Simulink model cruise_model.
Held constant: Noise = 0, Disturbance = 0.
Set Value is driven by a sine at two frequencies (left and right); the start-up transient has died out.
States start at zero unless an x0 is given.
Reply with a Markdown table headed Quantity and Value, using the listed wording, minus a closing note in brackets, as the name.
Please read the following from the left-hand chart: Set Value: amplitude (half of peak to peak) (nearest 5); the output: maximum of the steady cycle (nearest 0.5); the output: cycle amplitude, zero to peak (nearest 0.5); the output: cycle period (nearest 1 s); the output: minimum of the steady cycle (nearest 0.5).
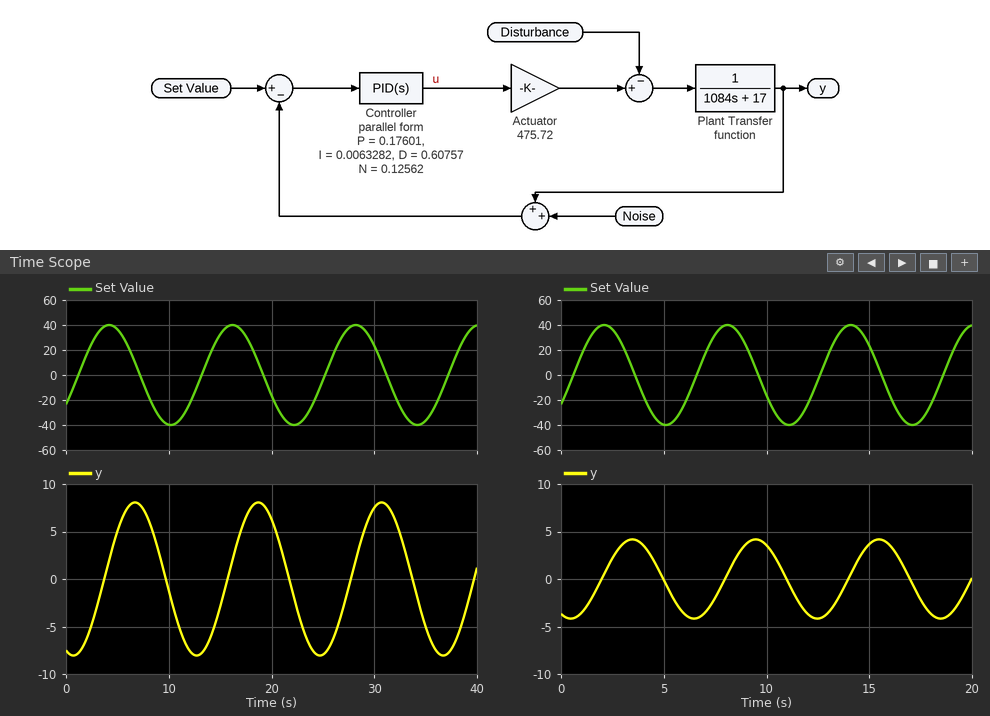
| Quantity | Value |
|---|---|
| Set Value: amplitude (half of peak to peak) | 40 |
| the output: maximum of the steady cycle | 8.0 |
| the output: cycle amplitude, zero to peak | 8.0 |
| the output: cycle period | 12 s |
| the output: minimum of the steady cycle | -8.0 |
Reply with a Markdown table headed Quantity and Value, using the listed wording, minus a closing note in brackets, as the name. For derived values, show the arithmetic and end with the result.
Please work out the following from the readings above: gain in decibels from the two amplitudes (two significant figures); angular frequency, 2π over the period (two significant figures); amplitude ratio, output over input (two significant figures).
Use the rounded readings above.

| Quantity | Value |
|---|---|
| gain in decibels from the two amplitudes | 20 log10(8 / 40) = -14 dB |
| angular frequency, 2π over the period | 2π / 12 = 0.52 rad/s |
| amplitude ratio, output over input | 8 / 40 = 0.20 |
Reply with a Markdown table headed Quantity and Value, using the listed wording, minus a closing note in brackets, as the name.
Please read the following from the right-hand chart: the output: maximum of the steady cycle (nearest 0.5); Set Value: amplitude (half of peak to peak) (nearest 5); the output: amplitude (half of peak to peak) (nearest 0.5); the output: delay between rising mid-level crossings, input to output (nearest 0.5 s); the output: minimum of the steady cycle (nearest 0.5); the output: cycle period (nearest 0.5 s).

| Quantity | Value |
|---|---|
| the output: maximum of the steady cycle | 4.0 |
| Set Value: amplitude (half of peak to peak) | 40 |
| the output: amplitude (half of peak to peak) | 4.0 |
| the output: delay between rising mid-level crossings, input to output | 1.5 s |
| the output: minimum of the steady cycle | -4.0 |
| the output: cycle period | 6.0 s |
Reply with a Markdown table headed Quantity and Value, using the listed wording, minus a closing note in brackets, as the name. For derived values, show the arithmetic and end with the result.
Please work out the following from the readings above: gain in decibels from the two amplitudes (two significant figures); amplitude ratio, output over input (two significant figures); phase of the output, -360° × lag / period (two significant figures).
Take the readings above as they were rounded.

| Quantity | Value |
|---|---|
| gain in decibels from the two amplitudes | 20 log10(4 / 40) = -20 dB |
| amplitude ratio, output over input | 4 / 40 = 0.10 |
| phase of the output, -360° × lag / period | -360 × 1.5 / 6 = -90° |
